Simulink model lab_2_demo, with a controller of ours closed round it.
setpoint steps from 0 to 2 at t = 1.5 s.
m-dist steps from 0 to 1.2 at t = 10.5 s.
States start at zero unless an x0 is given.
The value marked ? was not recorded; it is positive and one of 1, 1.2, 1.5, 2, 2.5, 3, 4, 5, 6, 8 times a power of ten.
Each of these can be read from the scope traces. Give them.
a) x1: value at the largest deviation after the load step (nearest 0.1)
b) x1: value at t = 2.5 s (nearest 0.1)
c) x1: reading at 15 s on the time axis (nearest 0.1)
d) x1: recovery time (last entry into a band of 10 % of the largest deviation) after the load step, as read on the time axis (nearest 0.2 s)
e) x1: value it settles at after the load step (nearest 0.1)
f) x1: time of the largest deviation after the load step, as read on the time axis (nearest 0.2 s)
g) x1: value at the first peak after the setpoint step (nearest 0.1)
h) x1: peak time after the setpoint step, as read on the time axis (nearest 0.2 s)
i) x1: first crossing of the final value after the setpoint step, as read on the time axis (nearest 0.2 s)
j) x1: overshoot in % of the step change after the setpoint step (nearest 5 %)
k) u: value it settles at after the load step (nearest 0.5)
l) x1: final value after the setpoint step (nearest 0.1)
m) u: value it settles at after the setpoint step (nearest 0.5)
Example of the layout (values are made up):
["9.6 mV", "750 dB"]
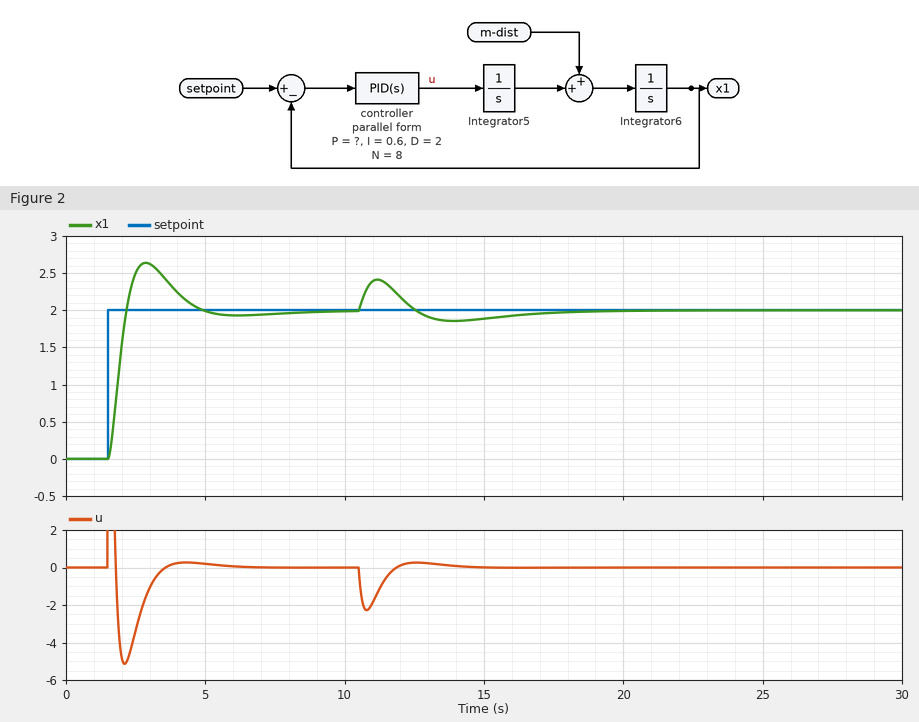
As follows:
["2.4", "2.5", "1.9", "17.0 s", "2.0", "11.2 s", "2.6", "2.8 s", "2.2 s", "30 %", "0.0", "2.0", "0.0"]
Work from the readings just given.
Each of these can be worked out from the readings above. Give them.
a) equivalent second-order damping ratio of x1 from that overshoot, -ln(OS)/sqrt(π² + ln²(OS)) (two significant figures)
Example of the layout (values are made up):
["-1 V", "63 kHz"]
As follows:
["0.36"]
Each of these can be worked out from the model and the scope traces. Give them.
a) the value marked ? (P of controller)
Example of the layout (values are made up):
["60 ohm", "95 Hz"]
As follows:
["2"]
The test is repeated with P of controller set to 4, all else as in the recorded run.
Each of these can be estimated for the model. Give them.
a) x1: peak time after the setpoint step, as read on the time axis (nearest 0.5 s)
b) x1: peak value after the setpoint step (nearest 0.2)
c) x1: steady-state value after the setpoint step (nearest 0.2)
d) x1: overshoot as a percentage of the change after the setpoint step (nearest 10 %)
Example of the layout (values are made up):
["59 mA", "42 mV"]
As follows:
["2.5 s", "2.8", "2.0", "40 %"]
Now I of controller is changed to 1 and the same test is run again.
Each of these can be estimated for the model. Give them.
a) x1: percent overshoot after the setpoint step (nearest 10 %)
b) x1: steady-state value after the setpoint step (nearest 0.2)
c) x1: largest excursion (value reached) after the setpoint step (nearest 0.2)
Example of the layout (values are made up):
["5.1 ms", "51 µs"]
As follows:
["40 %", "2.0", "2.8"]
